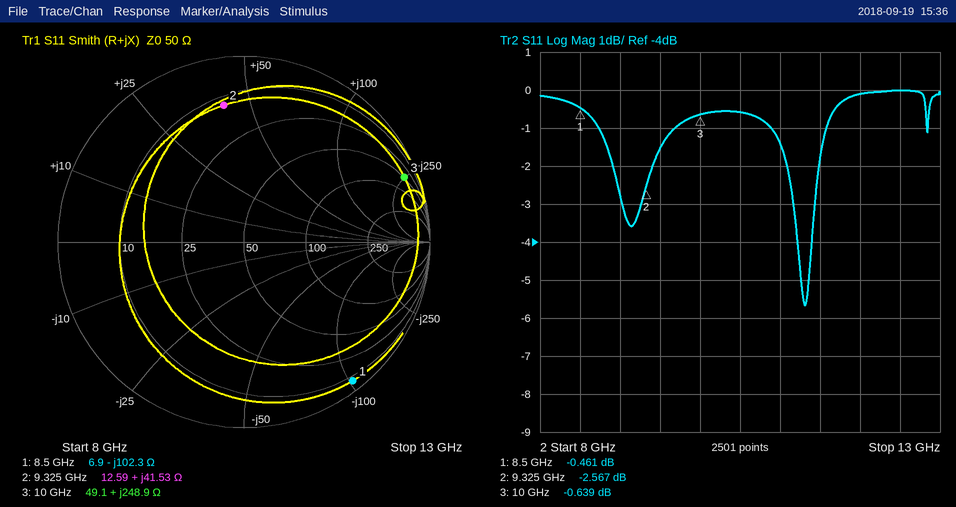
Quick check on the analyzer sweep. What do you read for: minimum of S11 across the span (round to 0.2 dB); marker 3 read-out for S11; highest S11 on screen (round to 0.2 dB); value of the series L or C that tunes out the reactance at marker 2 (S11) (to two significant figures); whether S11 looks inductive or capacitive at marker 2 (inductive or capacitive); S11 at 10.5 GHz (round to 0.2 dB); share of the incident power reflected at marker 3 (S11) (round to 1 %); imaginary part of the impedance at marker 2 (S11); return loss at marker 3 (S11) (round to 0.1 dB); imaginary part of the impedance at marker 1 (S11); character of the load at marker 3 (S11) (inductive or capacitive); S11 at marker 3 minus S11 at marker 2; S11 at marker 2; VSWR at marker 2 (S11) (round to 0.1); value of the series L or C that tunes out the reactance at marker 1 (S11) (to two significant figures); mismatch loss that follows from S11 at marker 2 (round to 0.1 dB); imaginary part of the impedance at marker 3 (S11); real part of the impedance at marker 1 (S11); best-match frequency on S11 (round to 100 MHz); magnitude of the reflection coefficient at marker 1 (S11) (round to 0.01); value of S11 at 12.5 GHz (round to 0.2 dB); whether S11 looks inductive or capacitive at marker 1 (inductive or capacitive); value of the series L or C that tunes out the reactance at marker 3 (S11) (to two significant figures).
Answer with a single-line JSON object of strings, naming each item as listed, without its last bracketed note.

{"minimum of S11 across the span": "-5.6 dB", "marker 3 read-out for S11": "-0.639 dB", "highest S11 on screen": "0.0 dB", "value of the series L or C that tunes out the reactance at marker 2 (S11)": "410 fF", "whether S11 looks inductive or capacitive at marker 2": "inductive", "S11 at 10.5 GHz": "-0.6 dB", "share of the incident power reflected at marker 3 (S11)": "86 %", "imaginary part of the impedance at marker 2": "+41.53 Ω", "return loss at marker 3 (S11)": "0.6 dB", "imaginary part of the impedance at marker 1": "-102.3 Ω", "character of the load at marker 3 (S11)": "inductive", "S11 at marker 3 minus S11 at marker 2": "1.928 dB", "S11 at marker 2": "-2.567 dB", "VSWR at marker 2 (S11)": "6.8", "value of the series L or C that tunes out the reactance at marker 1 (S11)": "1.9 nH", "mismatch loss that follows from S11 at marker 2": "3.5 dB", "imaginary part of the impedance at marker 3": "+248.9 Ω", "real part of the impedance at marker 1": "6.9 Ω", "best-match frequency on S11": "11.3 GHz", "magnitude of the reflection coefficient at marker 1 (S11)": "0.95", "value of S11 at 12.5 GHz": "0.0 dB", "whether S11 looks inductive or capacitive at marker 1": "capacitive", "value of the series L or C that tunes out the reactance at marker 3 (S11)": "64 fF"}
